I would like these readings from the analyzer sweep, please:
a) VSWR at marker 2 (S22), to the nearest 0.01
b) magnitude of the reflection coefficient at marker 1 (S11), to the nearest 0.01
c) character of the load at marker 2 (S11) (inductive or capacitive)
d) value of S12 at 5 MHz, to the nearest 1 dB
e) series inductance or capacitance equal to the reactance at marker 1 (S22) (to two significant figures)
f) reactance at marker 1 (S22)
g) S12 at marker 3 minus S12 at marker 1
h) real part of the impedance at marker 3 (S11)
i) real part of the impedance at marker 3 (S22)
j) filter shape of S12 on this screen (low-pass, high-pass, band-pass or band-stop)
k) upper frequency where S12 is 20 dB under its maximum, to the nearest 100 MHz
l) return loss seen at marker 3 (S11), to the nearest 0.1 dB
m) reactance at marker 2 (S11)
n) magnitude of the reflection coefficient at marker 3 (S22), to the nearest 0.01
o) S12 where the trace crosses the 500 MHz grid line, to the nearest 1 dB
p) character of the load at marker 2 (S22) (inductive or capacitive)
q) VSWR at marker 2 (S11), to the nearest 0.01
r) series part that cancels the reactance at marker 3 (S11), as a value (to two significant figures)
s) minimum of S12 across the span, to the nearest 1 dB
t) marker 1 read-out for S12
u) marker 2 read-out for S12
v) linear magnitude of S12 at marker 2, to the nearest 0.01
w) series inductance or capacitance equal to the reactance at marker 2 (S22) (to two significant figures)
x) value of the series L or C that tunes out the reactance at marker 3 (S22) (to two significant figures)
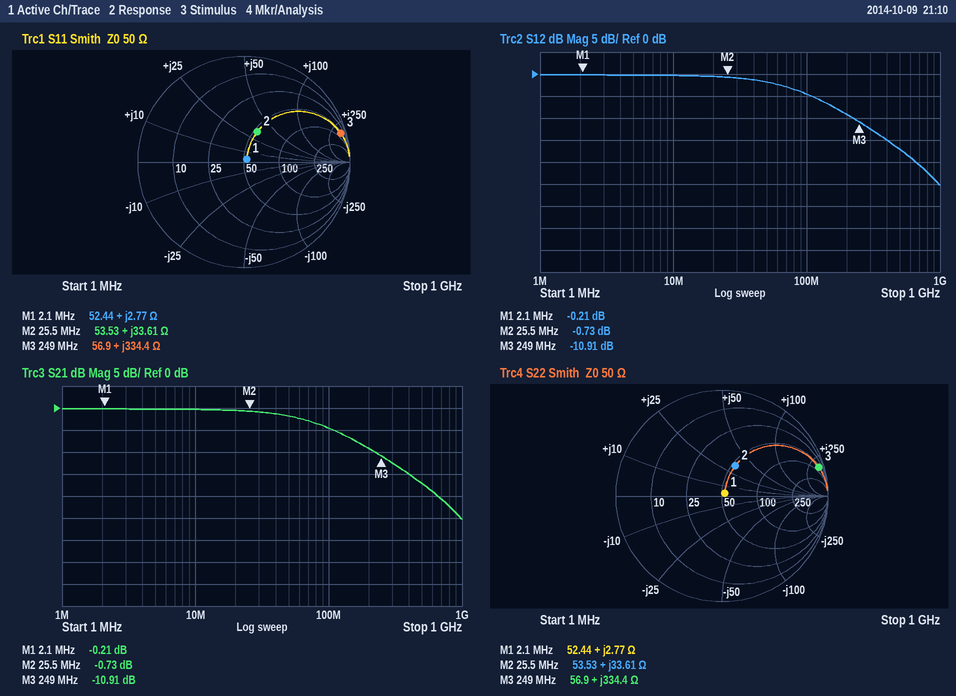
1.90
0.04
inductive
0 dB
210 nH
+2.77 Ω
-10.70 dB
56.9 Ω
56.9 Ω
low-pass
700 MHz
0.4 dB
+33.61 Ω
0.95
-17 dB
inductive
1.90
1.9 pF
-25 dB
-0.21 dB
-0.73 dB
0.92
210 nH
1.9 pF
